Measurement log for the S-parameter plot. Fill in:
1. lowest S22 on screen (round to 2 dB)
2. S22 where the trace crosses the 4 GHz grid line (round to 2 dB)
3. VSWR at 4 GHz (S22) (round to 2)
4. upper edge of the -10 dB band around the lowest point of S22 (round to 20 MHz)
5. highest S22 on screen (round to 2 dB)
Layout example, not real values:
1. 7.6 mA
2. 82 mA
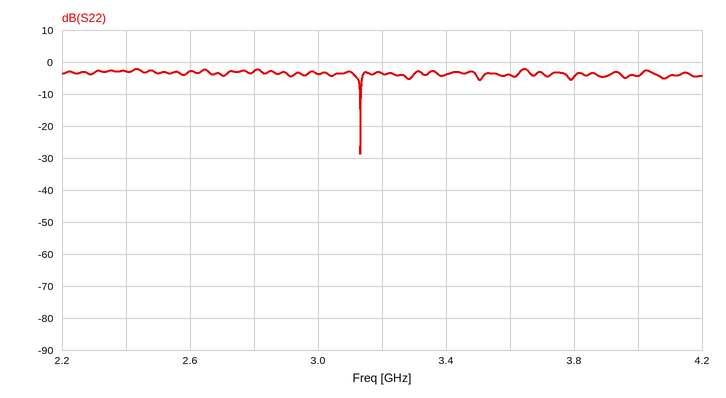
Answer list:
1. -28 dB
2. -4 dB
3. 4
4. 3.14 GHz
5. -2 dB
